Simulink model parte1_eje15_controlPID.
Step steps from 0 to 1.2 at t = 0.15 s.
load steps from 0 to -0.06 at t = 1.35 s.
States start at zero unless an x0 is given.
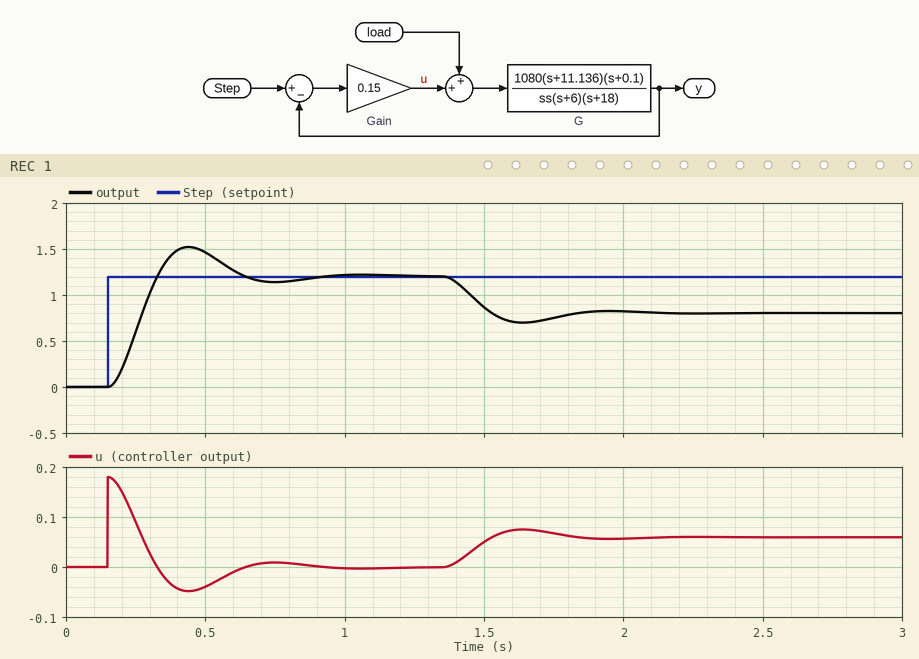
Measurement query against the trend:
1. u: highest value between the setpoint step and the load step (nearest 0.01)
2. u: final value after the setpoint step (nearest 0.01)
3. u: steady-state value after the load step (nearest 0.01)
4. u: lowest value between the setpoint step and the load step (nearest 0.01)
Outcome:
0.18
0.00
0.06
-0.05
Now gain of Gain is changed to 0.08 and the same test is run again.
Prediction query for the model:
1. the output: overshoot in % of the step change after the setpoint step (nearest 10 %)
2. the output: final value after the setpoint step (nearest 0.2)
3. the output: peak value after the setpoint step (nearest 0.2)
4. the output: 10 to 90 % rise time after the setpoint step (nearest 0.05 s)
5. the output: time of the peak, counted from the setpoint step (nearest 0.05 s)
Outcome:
20 %
1.2
1.4
0.20 s
0.45 s
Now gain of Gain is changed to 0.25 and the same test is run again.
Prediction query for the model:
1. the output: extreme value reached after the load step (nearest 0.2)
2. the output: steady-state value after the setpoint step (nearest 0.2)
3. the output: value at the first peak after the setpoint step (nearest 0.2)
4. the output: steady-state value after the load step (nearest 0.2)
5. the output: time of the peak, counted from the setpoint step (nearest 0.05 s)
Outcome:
0.8
1.2
1.6
1.0
0.20 s
